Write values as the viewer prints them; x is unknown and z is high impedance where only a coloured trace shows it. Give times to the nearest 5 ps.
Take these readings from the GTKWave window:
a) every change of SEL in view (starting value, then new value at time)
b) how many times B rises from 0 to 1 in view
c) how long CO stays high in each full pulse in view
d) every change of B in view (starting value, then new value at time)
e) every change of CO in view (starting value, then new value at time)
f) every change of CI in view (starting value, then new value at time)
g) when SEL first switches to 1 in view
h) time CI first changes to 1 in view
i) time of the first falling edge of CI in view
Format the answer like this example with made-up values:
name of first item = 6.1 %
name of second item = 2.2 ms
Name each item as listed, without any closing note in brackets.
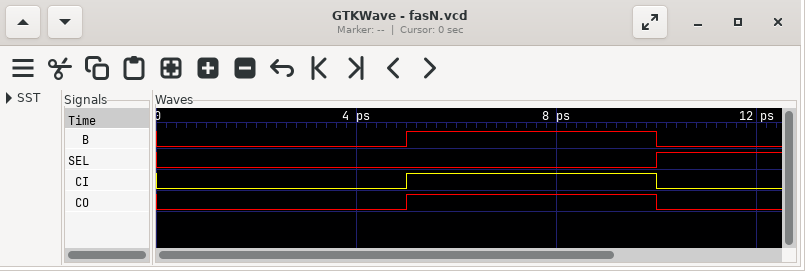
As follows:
every change of SEL in view = 0, 1 at 10 ps
how many times B rises from 0 to 1 in view = 1
how long CO stays high in each full pulse in view = 5 ps
every change of B in view = 0, 1 at 5 ps, 0 at 10 ps
every change of CO in view = 0, 1 at 5 ps, 0 at 10 ps
every change of CI in view = 0, 1 at 5 ps, 0 at 10 ps
when SEL first switches to 1 in view = 10 ps
time CI first changes to 1 in view = 5 ps
time of the first falling edge of CI in view = 10 ps
